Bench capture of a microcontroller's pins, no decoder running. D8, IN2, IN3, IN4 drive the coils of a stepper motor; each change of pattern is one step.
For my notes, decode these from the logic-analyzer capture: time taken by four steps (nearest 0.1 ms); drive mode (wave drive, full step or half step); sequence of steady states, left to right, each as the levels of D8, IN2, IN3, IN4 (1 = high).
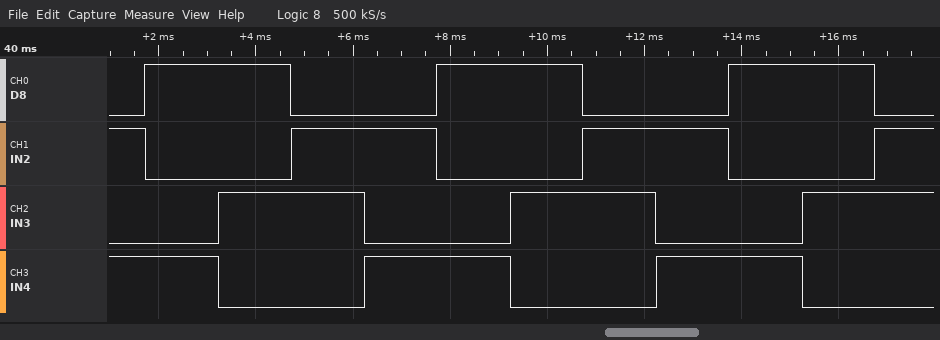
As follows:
6.0 ms
full step
0101 1001 1010 0110 0101 1001 1010 0110 0101 1001 1010 0110
